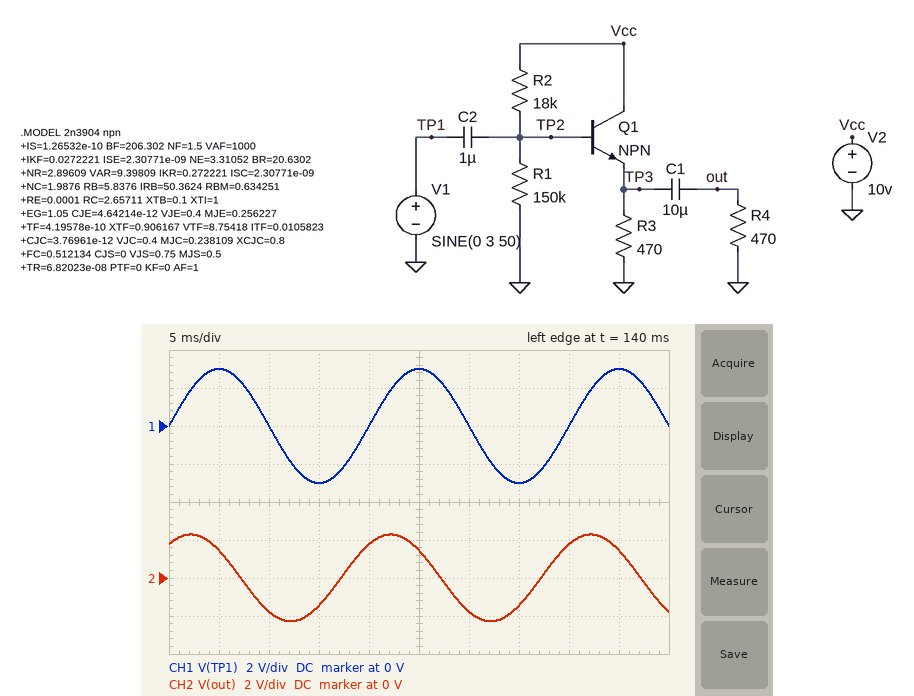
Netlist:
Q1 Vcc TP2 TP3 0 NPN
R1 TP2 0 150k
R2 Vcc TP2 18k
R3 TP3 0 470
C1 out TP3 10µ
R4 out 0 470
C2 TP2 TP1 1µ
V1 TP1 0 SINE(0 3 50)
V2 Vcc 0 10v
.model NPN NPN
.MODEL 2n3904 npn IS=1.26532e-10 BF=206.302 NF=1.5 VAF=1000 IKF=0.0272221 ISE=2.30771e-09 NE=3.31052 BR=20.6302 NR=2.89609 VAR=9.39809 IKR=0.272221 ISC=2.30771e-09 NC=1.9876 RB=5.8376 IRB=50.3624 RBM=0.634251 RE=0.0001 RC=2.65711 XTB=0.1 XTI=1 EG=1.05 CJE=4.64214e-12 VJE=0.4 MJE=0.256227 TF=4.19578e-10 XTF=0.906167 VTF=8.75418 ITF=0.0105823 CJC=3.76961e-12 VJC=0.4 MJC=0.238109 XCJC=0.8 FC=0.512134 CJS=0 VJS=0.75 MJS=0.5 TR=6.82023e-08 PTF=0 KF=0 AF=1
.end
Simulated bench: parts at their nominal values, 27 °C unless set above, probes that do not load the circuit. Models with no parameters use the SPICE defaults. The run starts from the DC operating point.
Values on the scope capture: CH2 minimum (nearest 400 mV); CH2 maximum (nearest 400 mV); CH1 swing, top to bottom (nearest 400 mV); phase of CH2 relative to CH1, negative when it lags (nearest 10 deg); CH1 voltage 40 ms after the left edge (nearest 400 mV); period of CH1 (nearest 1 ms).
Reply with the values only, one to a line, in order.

-2.4 V
2.4 V
6.0 V
50 deg
0 V
20 ms
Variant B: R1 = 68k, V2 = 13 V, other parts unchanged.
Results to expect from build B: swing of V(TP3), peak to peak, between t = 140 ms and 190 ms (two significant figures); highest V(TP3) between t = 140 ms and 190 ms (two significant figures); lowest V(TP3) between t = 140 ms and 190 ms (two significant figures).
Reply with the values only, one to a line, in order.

5.5 V
10 V
4.5 V
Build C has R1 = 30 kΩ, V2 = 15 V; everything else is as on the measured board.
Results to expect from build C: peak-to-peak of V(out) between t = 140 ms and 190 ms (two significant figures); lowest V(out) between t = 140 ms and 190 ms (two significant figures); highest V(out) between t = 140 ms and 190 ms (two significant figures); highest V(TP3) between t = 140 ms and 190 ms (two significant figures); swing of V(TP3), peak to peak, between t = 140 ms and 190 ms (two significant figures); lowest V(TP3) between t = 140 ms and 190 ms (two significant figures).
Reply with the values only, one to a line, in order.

4.5 V
-2.2 V
2.2 V
9.6 V
5.4 V
4.2 V
